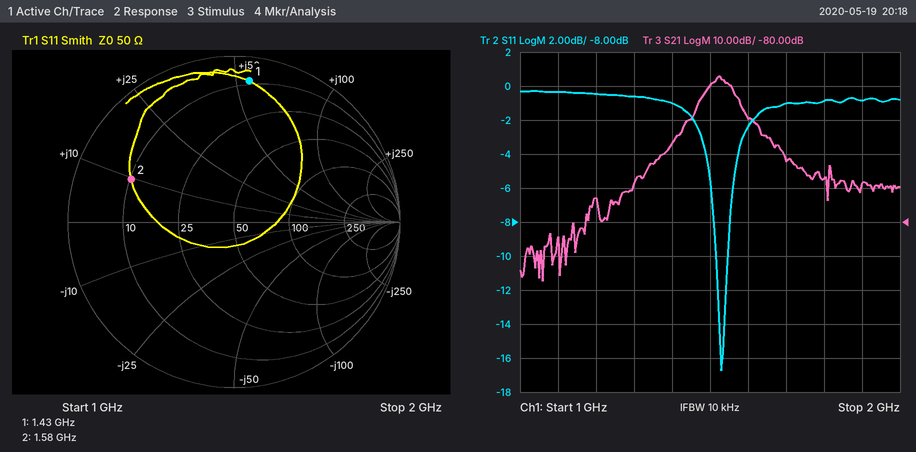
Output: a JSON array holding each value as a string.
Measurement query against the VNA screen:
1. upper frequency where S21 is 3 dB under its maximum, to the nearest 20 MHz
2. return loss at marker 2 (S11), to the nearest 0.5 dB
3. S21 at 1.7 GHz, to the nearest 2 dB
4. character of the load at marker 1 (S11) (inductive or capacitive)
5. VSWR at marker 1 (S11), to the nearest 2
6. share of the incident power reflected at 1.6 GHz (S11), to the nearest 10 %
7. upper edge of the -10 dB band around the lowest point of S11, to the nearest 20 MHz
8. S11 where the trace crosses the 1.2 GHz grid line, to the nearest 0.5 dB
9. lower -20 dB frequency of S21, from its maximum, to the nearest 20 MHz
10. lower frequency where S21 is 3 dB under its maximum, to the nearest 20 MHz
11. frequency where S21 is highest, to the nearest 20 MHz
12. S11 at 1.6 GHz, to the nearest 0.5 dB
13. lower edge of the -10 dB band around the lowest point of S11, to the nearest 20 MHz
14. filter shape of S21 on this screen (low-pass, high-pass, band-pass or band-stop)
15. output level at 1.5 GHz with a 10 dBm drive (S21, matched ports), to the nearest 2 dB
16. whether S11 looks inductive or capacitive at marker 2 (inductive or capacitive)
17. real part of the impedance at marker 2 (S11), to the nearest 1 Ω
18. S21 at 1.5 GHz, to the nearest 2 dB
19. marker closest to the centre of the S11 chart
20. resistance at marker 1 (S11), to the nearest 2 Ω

["1.56 GHz", "3.5 dB", "-62 dB", "inductive", "12", "60 %", "1.54 GHz", "-0.5 dB", "1.40 GHz", "1.50 GHz", "1.52 GHz", "-2.5 dB", "1.52 GHz", "band-pass", "-30 dBm", "inductive", "10 Ω", "-40 dB", "marker 2", "8 Ω"]
